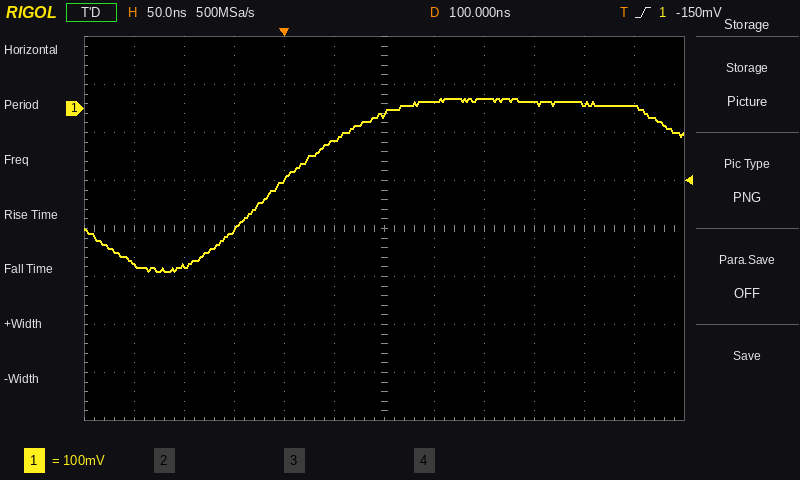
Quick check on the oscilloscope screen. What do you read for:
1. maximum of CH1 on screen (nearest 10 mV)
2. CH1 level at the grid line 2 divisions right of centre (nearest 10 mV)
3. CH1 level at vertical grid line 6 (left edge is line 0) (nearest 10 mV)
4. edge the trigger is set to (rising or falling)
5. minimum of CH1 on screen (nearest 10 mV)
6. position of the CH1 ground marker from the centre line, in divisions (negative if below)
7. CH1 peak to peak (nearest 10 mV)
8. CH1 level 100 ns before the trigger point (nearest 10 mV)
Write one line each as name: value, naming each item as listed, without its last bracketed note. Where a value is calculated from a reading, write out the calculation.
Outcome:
maximum of CH1 on screen: 20 mV
CH1 level at the grid line 2 divisions right of centre: 20 mV
CH1 level at vertical grid line 6 (left edge is line 0): -10 mV
edge the trigger is set to: rising
minimum of CH1 on screen: -340 mV
position of the CH1 ground marker from the centre line, in divisions: +2.5 div
CH1 peak to peak: 20 mV − (-340 mV) = 360 mV
CH1 level 100 ns before the trigger point: -330 mV
